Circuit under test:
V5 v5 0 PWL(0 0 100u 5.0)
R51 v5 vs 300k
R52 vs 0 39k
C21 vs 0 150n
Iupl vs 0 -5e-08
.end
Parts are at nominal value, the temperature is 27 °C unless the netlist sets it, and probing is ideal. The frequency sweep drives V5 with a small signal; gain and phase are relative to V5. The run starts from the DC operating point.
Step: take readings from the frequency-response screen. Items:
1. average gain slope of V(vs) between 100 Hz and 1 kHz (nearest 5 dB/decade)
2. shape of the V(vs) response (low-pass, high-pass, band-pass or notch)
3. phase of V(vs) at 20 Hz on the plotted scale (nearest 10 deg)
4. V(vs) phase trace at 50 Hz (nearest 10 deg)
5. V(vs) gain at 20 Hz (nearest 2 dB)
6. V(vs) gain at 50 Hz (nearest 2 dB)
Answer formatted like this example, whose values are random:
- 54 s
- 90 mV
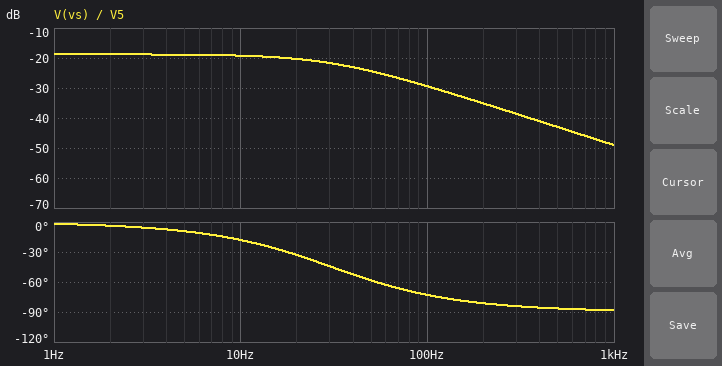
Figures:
- -20 dB/decade
- low-pass
- -30 deg
- -60 deg
- -20 dB
- -24 dB
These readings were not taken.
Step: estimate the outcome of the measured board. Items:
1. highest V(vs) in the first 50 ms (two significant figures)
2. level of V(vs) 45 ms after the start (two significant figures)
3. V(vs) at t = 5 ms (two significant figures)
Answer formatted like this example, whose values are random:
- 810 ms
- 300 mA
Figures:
- 580 mV
- 580 mV
- 360 mV
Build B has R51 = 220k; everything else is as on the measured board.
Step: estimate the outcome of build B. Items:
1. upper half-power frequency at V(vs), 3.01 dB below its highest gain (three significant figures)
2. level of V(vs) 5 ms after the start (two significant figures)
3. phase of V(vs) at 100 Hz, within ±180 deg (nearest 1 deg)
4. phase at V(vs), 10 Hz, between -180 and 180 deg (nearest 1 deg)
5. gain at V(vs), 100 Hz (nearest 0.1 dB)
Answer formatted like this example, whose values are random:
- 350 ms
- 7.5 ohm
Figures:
- 32.0 Hz
- 480 mV
- -72 deg
- -17 deg
- -26.8 dB
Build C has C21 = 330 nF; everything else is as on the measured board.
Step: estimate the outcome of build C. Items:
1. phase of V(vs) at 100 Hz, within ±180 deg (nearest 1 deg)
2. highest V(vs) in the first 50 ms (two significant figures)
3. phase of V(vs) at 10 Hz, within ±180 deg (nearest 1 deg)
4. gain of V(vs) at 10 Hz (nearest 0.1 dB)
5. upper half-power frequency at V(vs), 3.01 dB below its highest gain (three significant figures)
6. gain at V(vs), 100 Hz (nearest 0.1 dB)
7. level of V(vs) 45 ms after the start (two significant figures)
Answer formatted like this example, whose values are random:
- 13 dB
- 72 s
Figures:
- -82 deg
- 570 mV
- -36 deg
- -20.6 dB
- 14.0 Hz
- -36.0 dB
- 570 mV
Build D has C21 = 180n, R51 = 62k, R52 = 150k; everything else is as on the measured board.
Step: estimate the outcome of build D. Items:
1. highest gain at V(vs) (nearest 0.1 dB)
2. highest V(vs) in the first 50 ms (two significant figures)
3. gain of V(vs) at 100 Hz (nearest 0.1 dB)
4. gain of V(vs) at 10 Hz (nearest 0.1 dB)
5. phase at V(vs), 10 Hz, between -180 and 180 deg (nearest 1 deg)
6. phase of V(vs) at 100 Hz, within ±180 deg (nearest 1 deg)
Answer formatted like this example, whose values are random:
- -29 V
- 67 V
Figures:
- -3.0 dB
- 3.5 V
- -17.1 dB
- -4.0 dB
- -26 deg
- -79 deg
